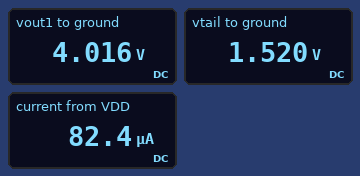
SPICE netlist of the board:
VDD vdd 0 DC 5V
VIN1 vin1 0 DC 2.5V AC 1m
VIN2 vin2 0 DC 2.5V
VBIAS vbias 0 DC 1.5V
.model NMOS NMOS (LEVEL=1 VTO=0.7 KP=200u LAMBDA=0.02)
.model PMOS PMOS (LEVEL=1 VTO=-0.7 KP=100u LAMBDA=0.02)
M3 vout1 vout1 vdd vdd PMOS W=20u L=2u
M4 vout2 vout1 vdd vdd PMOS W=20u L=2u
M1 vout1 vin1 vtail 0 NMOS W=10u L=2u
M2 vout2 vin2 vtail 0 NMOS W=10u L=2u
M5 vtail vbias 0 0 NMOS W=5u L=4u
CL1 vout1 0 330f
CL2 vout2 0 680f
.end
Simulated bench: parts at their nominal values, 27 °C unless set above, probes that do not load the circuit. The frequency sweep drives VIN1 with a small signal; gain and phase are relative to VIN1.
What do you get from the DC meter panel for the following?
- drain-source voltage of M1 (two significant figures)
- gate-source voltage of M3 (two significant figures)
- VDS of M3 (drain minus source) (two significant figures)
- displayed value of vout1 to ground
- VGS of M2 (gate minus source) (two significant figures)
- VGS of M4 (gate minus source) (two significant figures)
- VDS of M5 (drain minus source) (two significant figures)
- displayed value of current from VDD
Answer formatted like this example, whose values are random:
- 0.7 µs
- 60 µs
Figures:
- 2.5 V
- -980 mV
- -980 mV
- 4.016 V
- 980 mV
- -980 mV
- 1.5 V
- 82.4 µA
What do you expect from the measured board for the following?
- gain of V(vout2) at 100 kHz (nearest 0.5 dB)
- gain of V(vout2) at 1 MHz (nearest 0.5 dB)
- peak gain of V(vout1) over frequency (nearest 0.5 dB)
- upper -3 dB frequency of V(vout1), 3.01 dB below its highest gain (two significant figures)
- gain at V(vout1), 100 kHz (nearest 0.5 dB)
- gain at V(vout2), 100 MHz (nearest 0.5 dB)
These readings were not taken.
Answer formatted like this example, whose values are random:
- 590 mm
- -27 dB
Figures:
- 45.0 dB
- 36.0 dB
- -6.0 dB
- 140 MHz
- -11.0 dB
- -4.5 dB
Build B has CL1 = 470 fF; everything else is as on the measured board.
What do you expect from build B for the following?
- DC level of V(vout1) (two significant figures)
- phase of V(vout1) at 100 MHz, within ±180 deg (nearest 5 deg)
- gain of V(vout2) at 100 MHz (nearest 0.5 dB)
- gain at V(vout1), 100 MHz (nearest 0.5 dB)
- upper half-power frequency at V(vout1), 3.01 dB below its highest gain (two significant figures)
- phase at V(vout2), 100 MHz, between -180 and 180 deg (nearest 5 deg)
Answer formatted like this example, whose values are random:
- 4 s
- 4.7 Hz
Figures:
- 4.0 V
- 135 deg
- -5.5 dB
- -9.0 dB
- 99 MHz
- -110 deg
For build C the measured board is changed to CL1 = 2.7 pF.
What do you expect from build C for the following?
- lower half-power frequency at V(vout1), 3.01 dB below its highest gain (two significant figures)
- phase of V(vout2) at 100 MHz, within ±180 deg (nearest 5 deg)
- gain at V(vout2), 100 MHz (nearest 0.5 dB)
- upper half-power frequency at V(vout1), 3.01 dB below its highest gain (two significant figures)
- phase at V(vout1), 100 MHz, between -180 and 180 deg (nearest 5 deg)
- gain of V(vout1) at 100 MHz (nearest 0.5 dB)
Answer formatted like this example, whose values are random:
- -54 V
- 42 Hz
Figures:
- 250 kHz
- -100 deg
- -9.0 dB
- 18 MHz
- 100 deg
- -21.5 dB
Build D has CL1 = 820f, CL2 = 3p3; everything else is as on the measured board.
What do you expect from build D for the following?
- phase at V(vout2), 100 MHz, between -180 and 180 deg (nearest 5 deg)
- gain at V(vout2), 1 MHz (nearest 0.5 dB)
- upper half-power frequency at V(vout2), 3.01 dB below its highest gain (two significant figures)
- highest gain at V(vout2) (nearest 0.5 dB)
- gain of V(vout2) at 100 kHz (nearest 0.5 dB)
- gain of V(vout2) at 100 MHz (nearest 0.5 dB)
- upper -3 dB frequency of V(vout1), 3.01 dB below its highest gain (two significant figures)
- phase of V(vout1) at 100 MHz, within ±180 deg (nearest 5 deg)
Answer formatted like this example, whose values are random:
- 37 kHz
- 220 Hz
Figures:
- -110 deg
- 23.0 dB
- 77 kHz
- 45.5 dB
- 41.0 dB
- -20.5 dB
- 57 MHz
- 120 deg
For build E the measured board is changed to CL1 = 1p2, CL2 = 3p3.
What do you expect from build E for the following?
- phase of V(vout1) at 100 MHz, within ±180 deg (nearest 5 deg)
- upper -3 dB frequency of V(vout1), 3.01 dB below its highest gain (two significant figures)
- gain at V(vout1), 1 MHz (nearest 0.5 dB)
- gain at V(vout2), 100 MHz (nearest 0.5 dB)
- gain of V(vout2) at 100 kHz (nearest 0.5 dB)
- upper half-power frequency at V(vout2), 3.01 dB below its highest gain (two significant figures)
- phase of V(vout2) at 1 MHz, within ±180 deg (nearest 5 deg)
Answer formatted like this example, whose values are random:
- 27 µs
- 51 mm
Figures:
- 110 deg
- 39 MHz
- -6.0 dB
- -21.5 dB
- 41.0 dB
- 77 kHz
- -85 deg
